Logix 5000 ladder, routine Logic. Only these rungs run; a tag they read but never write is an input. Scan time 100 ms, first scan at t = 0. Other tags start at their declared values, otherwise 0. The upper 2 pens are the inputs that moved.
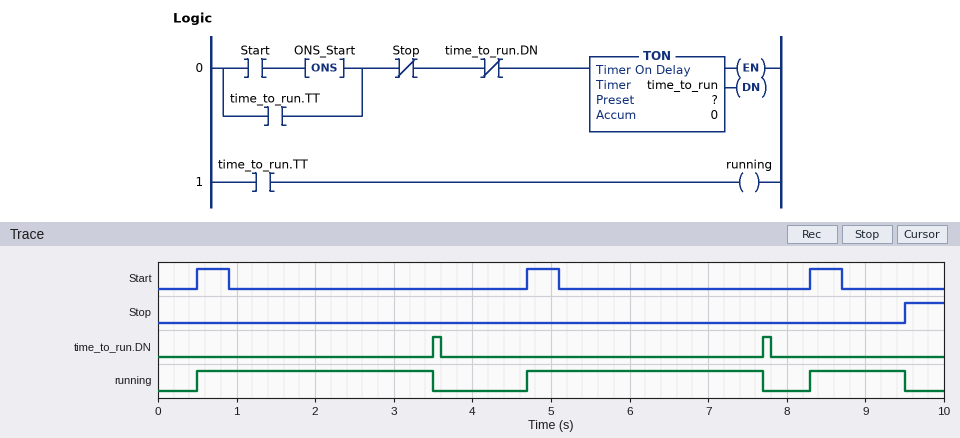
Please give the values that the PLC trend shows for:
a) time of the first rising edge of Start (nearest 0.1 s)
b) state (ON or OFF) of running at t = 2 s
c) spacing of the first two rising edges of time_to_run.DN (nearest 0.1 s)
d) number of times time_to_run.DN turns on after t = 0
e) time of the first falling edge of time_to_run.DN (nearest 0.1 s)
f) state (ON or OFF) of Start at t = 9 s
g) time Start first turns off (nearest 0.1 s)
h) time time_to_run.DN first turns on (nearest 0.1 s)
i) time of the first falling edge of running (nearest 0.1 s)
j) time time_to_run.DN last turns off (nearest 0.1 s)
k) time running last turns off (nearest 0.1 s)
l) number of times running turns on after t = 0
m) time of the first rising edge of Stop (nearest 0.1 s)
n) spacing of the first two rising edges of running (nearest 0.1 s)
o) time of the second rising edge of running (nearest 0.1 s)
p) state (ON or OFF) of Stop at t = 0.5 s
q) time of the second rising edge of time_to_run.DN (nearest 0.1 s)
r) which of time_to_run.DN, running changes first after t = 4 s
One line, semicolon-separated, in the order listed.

0.5 s; ON; 4.2 s; 2; 3.6 s; OFF; 0.9 s; 3.5 s; 3.5 s; 7.8 s; 9.5 s; 3; 9.5 s; 4.2 s; 4.7 s; OFF; 7.7 s; running
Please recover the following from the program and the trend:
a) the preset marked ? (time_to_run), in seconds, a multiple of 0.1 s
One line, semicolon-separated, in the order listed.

3.0 s
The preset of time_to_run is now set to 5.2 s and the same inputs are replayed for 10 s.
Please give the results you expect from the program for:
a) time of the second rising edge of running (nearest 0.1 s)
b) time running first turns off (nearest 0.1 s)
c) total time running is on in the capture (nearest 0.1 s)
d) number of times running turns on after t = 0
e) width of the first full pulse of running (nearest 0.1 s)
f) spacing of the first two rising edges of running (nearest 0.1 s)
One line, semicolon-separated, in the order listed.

8.3 s; 5.7 s; 6.4 s; 2; 5.2 s; 7.8 s
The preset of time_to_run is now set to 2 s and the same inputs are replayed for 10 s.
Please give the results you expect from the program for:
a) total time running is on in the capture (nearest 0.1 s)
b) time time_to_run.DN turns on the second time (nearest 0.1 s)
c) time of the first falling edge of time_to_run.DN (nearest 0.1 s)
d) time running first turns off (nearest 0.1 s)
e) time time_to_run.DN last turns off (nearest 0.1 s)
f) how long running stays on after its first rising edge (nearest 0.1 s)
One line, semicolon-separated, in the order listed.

5.2 s; 6.7 s; 2.6 s; 2.5 s; 6.8 s; 2.0 s
